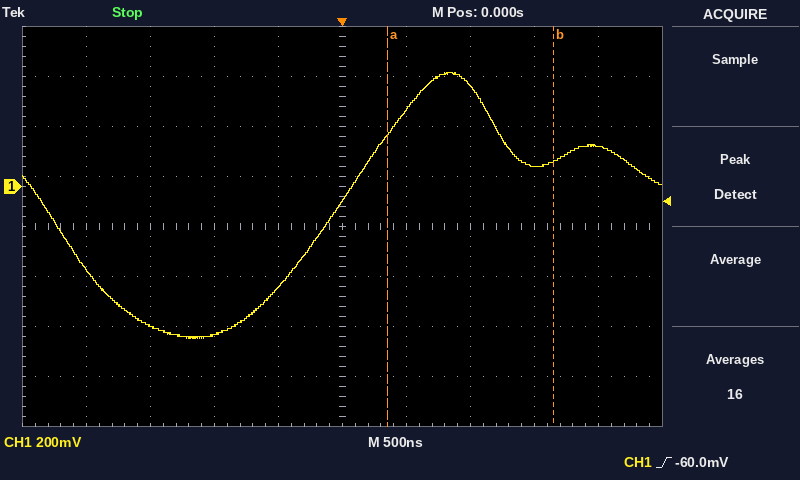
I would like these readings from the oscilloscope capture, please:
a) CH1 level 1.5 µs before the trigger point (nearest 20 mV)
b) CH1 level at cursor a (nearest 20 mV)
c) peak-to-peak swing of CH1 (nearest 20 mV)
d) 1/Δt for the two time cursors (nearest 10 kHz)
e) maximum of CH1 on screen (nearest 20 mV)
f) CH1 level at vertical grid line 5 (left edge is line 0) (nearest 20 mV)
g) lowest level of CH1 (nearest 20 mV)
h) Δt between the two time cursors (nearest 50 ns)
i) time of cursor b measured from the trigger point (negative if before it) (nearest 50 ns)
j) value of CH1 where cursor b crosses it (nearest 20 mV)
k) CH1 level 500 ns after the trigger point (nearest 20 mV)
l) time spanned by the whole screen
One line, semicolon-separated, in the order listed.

-560 mV; 200 mV; 1.06 V; 770 kHz; 460 mV; -60 mV; -600 mV; 1.30 µs; +1.65 µs; 100 mV; 300 mV; 5 µs
